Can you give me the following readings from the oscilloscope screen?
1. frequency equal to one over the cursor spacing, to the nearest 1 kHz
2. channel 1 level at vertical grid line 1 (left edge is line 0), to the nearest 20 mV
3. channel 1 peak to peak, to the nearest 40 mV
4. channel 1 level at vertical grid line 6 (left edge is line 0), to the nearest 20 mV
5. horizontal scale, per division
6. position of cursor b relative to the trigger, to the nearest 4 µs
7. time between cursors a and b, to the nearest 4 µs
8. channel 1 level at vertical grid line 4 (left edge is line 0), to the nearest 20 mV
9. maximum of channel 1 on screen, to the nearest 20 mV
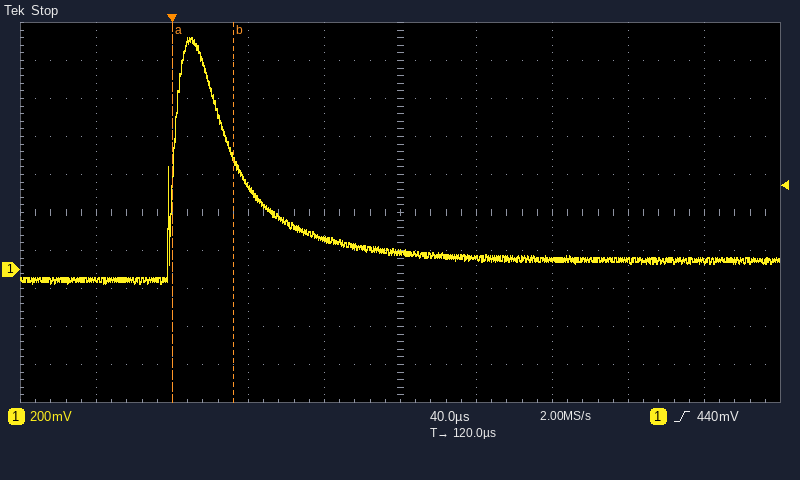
31 kHz
-60 mV
1.28 V
60 mV
40 µs
+32 µs
32 µs
160 mV
1.22 V
